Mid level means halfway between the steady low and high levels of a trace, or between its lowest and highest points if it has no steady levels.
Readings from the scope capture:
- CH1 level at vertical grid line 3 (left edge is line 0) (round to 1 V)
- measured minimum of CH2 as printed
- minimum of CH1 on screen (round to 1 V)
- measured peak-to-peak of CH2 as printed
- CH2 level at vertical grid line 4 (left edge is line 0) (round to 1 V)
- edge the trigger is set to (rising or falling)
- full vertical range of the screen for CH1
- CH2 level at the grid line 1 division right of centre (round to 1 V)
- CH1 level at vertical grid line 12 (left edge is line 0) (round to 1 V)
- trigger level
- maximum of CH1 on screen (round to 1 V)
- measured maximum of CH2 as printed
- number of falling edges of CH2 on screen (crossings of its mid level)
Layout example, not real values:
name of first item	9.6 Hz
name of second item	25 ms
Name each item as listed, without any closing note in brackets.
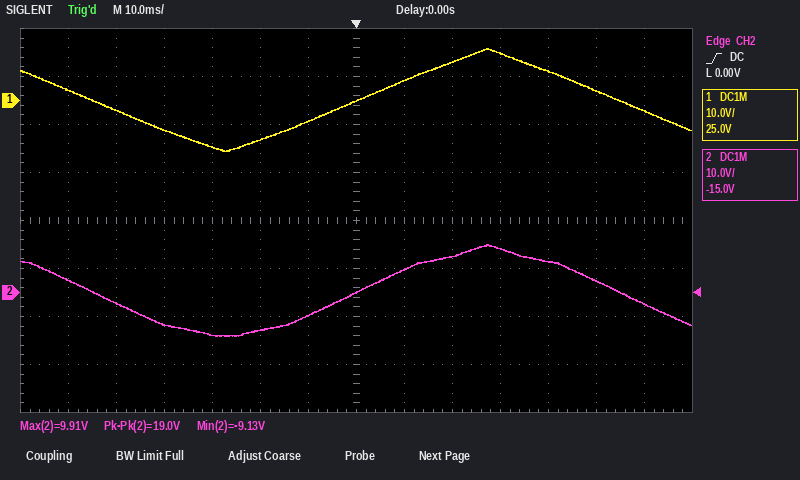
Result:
CH1 level at vertical grid line 3 (left edge is line 0)	-6 V
measured minimum of CH2 as printed	-9.13 V
minimum of CH1 on screen	-11 V
measured peak-to-peak of CH2 as printed	19.0 V
CH2 level at vertical grid line 4 (left edge is line 0)	-9 V
edge the trigger is set to	rising
full vertical range of the screen for CH1	80 V
CH2 level at the grid line 1 division right of centre	5 V
CH1 level at vertical grid line 12 (left edge is line 0)	2 V
trigger level	0.00 V
maximum of CH1 on screen	11 V
measured maximum of CH2 as printed	9.91 V
number of falling edges of CH2 on screen	2
